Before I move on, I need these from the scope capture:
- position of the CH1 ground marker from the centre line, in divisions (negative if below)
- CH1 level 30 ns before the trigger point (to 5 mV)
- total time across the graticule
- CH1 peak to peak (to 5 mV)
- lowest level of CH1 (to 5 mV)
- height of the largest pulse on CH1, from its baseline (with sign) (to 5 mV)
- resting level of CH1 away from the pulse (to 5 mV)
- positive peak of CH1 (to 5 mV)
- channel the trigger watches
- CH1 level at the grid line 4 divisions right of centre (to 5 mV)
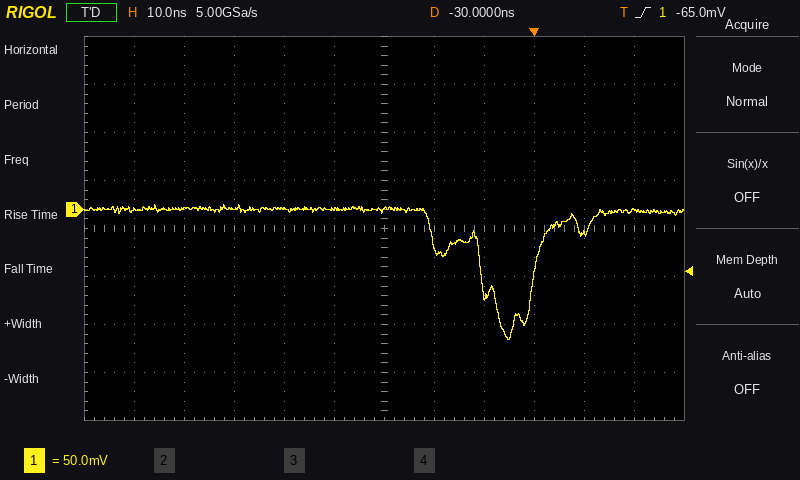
+0.4 div
0 mV
120 ns
140 mV
-135 mV
-135 mV
0 mV
5 mV
CH1
-25 mV
